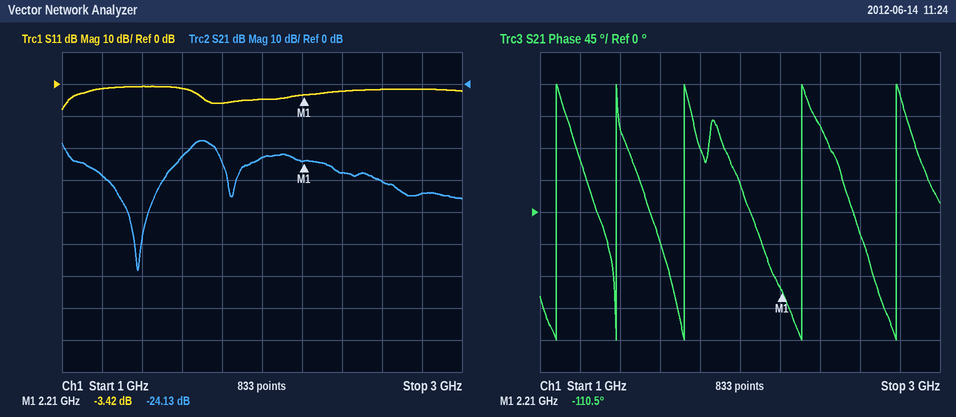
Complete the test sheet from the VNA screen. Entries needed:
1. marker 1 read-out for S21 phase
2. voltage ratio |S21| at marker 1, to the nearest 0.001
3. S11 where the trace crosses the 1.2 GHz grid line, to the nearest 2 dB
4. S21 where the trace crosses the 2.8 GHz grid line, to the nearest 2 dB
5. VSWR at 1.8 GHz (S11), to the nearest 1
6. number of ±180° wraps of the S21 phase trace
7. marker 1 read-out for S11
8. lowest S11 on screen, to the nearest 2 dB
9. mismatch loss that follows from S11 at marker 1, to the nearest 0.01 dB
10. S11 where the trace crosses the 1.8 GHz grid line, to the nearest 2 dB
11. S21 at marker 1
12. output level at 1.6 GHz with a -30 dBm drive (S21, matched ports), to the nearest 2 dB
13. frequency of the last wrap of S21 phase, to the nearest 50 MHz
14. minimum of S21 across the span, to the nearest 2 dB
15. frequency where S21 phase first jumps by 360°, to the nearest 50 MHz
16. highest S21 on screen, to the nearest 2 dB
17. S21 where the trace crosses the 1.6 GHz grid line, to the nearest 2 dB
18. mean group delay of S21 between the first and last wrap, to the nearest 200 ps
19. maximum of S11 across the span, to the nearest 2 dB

-110.5°
0.062
-2 dB
-34 dB
3
5
-3.42 dB
-8 dB
2.64 dB
-6 dB
-24.13 dB
-52 dBm
2.80 GHz
-58 dB
1.10 GHz
-18 dB
-22 dB
2.4 ns
0 dB
